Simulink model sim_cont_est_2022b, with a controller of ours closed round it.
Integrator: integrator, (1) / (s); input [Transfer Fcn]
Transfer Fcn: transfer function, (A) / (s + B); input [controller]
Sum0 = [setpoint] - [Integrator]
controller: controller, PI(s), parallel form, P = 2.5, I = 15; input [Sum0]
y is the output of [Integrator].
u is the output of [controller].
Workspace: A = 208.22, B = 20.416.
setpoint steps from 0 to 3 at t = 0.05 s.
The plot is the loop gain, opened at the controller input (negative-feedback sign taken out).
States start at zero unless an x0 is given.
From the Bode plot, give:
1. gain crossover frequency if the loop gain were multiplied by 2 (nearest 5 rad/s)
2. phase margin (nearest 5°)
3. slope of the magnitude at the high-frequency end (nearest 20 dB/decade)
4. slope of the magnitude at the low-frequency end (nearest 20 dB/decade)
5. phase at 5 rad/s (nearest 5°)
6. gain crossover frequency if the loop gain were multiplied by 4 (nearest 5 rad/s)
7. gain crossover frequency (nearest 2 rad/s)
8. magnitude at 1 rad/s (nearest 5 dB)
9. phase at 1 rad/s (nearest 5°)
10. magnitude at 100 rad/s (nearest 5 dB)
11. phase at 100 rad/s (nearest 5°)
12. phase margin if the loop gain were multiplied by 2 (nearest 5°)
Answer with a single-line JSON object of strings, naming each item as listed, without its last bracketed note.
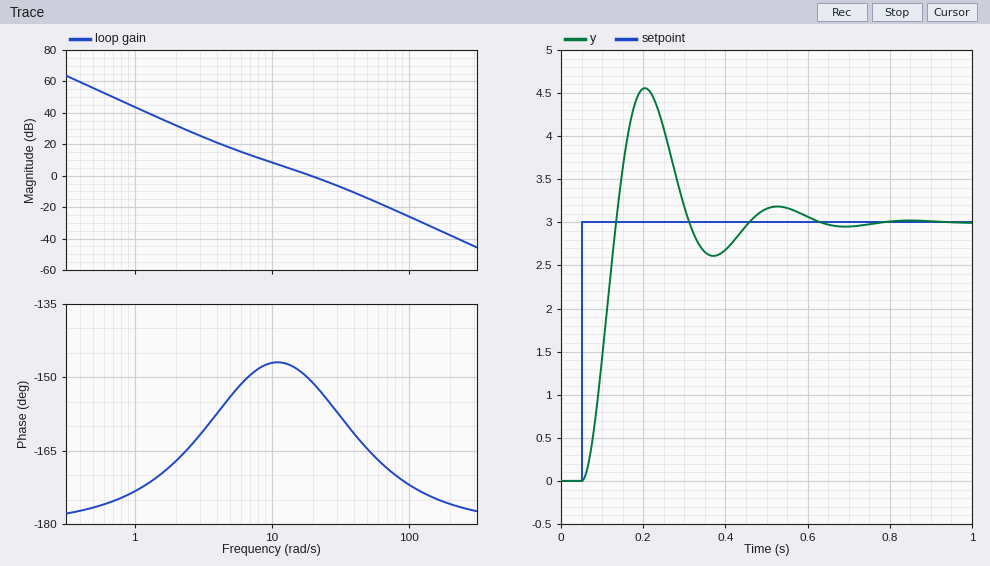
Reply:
{"gain crossover frequency if the loop gain were multiplied by 2": "30 rad/s", "phase margin": "30°", "slope of the magnitude at the high-frequency end": "-40 dB/decade", "slope of the magnitude at the low-frequency end": "-40 dB/decade", "phase at 5 rad/s": "-155°", "gain crossover frequency if the loop gain were multiplied by 4": "45 rad/s", "gain crossover frequency": "20 rad/s", "magnitude at 1 rad/s": "45 dB", "phase at 1 rad/s": "-175°", "magnitude at 100 rad/s": "-25 dB", "phase at 100 rad/s": "-170°", "phase margin if the loop gain were multiplied by 2": "25°"}
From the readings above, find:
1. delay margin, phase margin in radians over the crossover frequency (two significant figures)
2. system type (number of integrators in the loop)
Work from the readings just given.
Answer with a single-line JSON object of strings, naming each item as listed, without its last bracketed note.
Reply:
{"delay margin, phase margin in radians over the crossover frequency": "0.026 s", "system type": "2"}
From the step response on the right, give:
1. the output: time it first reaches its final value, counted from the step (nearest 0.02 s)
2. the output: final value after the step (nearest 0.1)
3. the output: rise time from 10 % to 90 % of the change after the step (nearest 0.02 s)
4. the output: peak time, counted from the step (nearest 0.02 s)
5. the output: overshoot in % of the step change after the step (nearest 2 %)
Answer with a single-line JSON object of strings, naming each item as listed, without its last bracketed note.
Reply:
{"the output: time it first reaches its final value, counted from the step": "0.08 s", "the output: final value after the step": "3.0", "the output: rise time from 10 % to 90 % of the change after the step": "0.06 s", "the output: peak time, counted from the step": "0.16 s", "the output: overshoot in % of the step change after the step": "52 %"}
